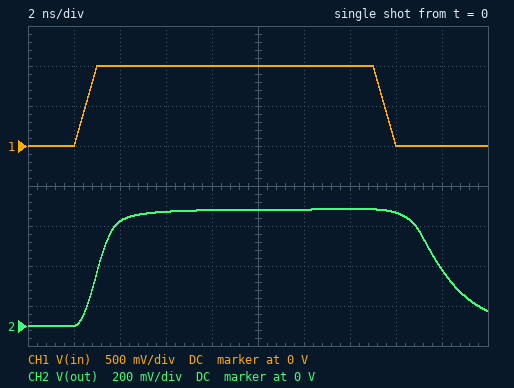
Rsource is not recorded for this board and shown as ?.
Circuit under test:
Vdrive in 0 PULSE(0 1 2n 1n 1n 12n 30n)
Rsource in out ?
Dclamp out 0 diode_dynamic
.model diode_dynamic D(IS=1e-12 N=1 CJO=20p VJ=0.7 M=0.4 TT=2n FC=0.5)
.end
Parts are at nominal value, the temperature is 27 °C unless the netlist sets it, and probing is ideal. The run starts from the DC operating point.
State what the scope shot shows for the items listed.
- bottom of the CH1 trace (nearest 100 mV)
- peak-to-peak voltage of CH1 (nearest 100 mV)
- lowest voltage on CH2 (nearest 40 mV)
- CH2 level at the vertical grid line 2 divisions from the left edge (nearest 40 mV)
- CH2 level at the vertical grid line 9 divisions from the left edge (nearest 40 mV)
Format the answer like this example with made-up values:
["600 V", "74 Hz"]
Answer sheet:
["0 V", "1.0 V", "0 V", "520 mV", "280 mV"]
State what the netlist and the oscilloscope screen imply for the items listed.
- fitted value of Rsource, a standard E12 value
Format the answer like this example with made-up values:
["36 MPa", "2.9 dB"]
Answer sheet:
["68 Ω"]
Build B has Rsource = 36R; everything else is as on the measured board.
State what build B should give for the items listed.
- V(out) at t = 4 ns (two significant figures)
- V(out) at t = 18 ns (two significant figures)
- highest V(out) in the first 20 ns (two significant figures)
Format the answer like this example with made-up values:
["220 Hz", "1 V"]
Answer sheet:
["570 mV", "130 mV", "600 mV"]
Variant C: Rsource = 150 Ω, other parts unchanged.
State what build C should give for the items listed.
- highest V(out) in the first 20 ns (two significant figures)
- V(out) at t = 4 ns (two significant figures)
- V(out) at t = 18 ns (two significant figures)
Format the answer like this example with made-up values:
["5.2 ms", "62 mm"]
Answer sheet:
["560 mV", "350 mV", "410 mV"]
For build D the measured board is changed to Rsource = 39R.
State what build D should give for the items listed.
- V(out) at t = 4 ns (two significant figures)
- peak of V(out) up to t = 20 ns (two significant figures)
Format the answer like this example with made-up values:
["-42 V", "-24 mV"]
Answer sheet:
["560 mV", "600 mV"]
